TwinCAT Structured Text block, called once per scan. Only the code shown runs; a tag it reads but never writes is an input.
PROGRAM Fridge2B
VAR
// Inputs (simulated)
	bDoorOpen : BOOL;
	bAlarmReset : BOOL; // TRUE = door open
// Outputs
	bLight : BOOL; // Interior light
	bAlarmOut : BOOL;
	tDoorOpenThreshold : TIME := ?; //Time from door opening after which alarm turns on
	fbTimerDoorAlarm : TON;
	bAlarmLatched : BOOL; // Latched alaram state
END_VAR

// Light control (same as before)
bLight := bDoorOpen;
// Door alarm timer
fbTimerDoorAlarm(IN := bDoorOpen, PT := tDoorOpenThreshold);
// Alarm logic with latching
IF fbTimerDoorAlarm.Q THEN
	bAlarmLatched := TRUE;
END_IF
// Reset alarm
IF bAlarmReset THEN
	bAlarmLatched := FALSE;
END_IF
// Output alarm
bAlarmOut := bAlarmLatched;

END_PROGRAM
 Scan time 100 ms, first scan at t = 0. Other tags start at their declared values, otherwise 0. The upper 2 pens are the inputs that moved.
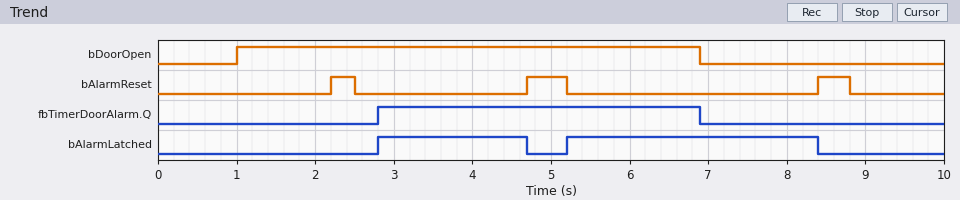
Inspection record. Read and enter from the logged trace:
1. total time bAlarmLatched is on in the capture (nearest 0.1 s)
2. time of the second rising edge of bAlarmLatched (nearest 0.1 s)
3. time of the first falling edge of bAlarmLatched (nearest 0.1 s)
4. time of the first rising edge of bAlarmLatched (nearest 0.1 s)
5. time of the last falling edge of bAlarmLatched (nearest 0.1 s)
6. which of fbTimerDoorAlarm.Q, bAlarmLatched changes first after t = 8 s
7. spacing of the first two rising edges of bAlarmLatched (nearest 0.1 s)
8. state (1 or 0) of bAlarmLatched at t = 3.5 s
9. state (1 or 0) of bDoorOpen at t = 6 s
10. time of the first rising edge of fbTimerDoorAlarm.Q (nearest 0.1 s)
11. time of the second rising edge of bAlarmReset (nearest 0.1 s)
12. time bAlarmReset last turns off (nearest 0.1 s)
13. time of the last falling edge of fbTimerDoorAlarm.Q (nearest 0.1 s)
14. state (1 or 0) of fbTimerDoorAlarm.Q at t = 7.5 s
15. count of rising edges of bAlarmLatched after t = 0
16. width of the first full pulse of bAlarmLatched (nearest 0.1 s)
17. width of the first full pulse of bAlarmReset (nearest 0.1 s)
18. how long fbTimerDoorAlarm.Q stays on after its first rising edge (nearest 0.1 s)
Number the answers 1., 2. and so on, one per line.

1. 5.1 s
2. 5.2 s
3. 4.7 s
4. 2.8 s
5. 8.4 s
6. bAlarmLatched
7. 2.4 s
8. 1
9. 1
10. 2.8 s
11. 4.7 s
12. 8.8 s
13. 6.9 s
14. 0
15. 2
16. 1.9 s
17. 0.3 s
18. 4.1 s
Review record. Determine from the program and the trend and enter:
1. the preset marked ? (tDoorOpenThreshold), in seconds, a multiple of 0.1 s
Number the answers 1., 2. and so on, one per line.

1. 1.8 s
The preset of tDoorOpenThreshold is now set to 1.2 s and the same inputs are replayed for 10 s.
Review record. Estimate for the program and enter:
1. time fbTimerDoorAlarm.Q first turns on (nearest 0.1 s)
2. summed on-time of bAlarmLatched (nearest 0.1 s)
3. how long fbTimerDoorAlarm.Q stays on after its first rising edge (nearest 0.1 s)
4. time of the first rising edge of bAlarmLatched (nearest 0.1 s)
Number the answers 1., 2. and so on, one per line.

1. 2.2 s
2. 5.4 s
3. 4.7 s
4. 2.5 s
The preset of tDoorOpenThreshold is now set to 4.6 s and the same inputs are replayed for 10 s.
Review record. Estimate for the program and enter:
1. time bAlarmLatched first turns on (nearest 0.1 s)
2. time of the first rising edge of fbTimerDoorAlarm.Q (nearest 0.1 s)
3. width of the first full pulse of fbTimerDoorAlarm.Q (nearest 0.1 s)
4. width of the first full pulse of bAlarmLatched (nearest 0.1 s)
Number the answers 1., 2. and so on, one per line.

1. 5.6 s
2. 5.6 s
3. 1.3 s
4. 2.8 s
